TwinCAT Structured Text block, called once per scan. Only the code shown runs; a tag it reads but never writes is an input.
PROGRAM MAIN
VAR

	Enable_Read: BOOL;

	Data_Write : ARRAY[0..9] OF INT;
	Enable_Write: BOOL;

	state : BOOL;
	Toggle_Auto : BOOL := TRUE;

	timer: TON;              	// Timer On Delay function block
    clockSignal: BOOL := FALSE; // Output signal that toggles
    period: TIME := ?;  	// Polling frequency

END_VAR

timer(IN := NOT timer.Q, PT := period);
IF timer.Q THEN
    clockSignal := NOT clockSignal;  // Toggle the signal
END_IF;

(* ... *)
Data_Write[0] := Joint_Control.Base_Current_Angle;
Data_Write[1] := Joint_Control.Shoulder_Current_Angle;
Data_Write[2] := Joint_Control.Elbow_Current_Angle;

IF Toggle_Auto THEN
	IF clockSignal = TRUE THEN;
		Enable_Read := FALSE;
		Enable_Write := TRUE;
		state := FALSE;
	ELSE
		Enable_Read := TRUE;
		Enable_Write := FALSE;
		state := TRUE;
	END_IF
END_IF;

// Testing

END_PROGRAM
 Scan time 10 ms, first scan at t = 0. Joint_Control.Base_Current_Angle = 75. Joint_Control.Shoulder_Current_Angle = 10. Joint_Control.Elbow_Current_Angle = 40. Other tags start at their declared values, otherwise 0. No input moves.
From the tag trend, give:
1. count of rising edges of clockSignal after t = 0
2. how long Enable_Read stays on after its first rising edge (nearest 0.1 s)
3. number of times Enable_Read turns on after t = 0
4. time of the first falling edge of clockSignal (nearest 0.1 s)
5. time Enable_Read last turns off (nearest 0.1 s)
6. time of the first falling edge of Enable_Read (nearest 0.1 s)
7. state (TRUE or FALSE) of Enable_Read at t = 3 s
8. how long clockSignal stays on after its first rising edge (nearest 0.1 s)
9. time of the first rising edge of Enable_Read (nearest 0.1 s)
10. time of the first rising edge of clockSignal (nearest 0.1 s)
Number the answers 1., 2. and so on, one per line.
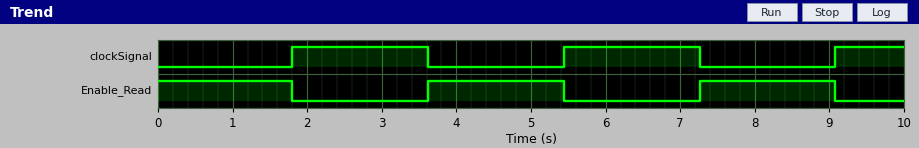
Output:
1. 3
2. 1.8 s
3. 2
4. 3.6 s
5. 9.1 s
6. 1.8 s
7. FALSE
8. 1.8 s
9. 3.6 s
10. 1.8 s
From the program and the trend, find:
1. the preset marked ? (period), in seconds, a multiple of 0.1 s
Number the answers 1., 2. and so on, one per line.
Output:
1. 1.8 s
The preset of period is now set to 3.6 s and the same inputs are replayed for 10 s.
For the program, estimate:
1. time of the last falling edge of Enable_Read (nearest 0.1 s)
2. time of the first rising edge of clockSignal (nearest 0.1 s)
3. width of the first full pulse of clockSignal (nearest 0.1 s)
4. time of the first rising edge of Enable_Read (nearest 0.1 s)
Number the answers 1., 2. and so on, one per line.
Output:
1. 3.6 s
2. 3.6 s
3. 3.6 s
4. 7.2 s
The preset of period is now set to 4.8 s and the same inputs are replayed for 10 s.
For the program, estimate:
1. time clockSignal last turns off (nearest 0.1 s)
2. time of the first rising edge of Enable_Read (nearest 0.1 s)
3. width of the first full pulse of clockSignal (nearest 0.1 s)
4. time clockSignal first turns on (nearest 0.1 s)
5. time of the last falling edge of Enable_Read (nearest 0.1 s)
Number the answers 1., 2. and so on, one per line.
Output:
1. 9.6 s
2. 9.6 s
3. 4.8 s
4. 4.8 s
5. 4.8 s
